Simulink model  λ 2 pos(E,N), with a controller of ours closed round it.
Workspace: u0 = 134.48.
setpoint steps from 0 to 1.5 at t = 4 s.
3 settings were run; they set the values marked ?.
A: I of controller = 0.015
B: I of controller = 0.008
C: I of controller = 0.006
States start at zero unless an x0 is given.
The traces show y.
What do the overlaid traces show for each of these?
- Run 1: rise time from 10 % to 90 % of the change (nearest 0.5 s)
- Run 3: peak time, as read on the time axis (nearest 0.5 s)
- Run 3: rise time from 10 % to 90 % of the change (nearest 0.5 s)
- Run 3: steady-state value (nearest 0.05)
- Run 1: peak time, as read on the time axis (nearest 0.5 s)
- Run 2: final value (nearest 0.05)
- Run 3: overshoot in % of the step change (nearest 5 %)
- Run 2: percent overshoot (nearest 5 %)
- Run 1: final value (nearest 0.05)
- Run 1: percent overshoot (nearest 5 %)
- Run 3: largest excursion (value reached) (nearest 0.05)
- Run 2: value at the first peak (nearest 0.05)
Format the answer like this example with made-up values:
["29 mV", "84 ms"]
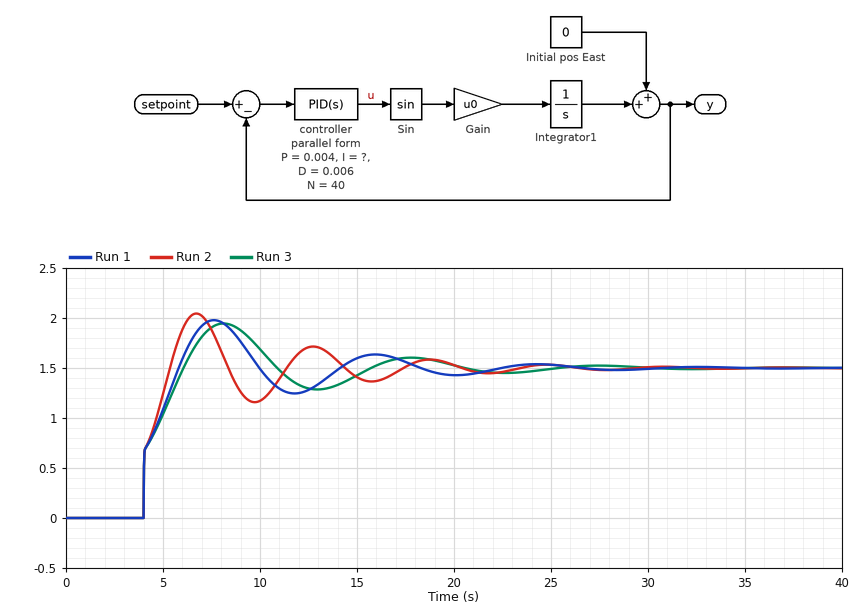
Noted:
["1.5 s", "8.0 s", "1.5 s", "1.50", "7.5 s", "1.50", "30 %", "35 %", "1.50", "30 %", "1.95", "2.05"]
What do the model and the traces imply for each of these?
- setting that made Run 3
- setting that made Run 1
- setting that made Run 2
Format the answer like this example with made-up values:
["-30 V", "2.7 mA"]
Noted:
["C", "B", "A"]
